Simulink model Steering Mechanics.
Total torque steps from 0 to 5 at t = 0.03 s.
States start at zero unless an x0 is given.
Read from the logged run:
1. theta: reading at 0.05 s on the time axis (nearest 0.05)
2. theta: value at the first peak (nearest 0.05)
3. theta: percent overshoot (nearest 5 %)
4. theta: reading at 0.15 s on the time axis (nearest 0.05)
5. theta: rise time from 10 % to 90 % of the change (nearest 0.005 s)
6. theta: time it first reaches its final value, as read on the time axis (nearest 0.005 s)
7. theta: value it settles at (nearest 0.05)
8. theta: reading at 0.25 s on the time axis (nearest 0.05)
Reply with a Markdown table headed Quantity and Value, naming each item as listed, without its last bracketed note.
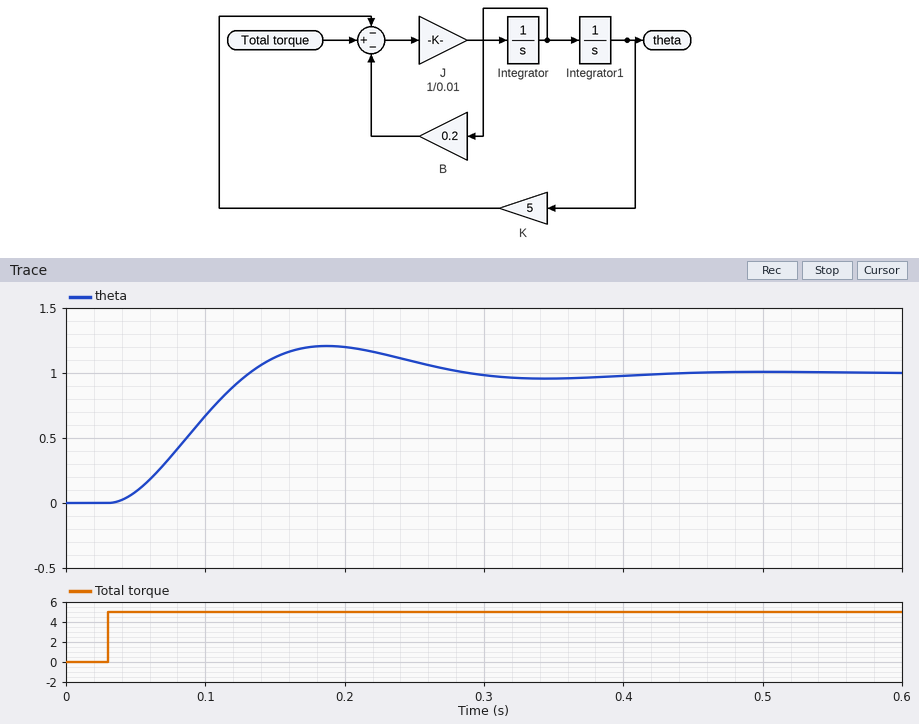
| Quantity | Value |
|---|---|
| theta: reading at 0.05 s on the time axis | 0.10 |
| theta: value at the first peak | 1.20 |
| theta: percent overshoot | 20 % |
| theta: reading at 0.15 s on the time axis | 1.10 |
| theta: rise time from 10 % to 90 % of the change | 0.070 s |
| theta: time it first reaches its final value, as read on the time axis | 0.130 s |
| theta: value it settles at | 1.00 |
| theta: reading at 0.25 s on the time axis | 1.10 |
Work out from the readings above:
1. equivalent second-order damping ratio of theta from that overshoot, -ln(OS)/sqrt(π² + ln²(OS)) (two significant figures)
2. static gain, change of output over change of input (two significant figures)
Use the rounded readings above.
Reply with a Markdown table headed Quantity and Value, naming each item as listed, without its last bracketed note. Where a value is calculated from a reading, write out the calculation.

| Quantity | Value |
|---|---|
| equivalent second-order damping ratio of theta from that overshoot, -ln(OS)/sqrt(π² + ln²(OS)) | ln(0.2) = -1.609; 1.609 / sqrt(9.870 + 2.590) = 0.46 |
| static gain, change of output over change of input | (1 - 0) / (5 - 0) = 0.20 |
